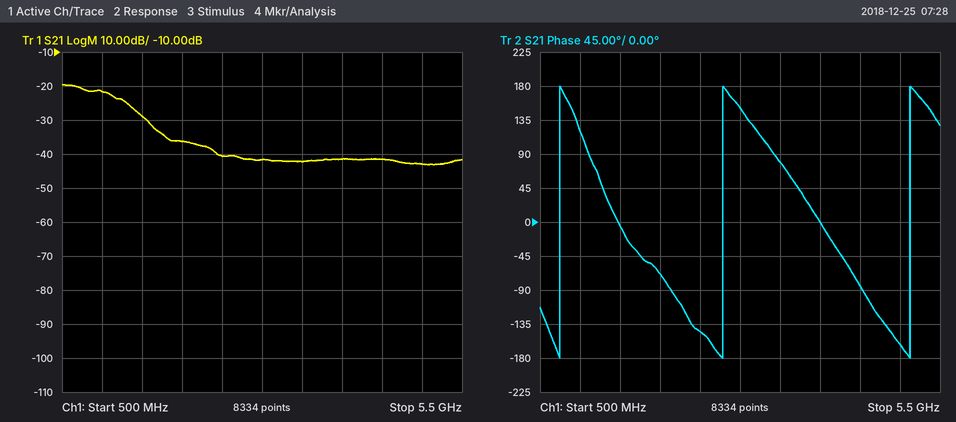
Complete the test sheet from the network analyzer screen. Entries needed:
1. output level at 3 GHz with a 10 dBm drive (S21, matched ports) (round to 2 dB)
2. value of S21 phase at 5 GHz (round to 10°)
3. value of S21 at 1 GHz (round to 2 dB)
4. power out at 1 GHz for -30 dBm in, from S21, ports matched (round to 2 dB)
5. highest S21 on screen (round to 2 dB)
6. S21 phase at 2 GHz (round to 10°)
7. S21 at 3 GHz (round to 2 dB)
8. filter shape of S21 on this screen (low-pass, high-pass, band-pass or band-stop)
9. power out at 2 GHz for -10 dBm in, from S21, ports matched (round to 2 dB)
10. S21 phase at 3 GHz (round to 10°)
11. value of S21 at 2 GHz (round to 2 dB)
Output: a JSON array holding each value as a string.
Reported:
["-32 dBm", "-160°", "-22 dB", "-52 dBm", "-20 dB", "-70°", "-42 dB", "low-pass", "-46 dBm", "150°", "-36 dB"]
